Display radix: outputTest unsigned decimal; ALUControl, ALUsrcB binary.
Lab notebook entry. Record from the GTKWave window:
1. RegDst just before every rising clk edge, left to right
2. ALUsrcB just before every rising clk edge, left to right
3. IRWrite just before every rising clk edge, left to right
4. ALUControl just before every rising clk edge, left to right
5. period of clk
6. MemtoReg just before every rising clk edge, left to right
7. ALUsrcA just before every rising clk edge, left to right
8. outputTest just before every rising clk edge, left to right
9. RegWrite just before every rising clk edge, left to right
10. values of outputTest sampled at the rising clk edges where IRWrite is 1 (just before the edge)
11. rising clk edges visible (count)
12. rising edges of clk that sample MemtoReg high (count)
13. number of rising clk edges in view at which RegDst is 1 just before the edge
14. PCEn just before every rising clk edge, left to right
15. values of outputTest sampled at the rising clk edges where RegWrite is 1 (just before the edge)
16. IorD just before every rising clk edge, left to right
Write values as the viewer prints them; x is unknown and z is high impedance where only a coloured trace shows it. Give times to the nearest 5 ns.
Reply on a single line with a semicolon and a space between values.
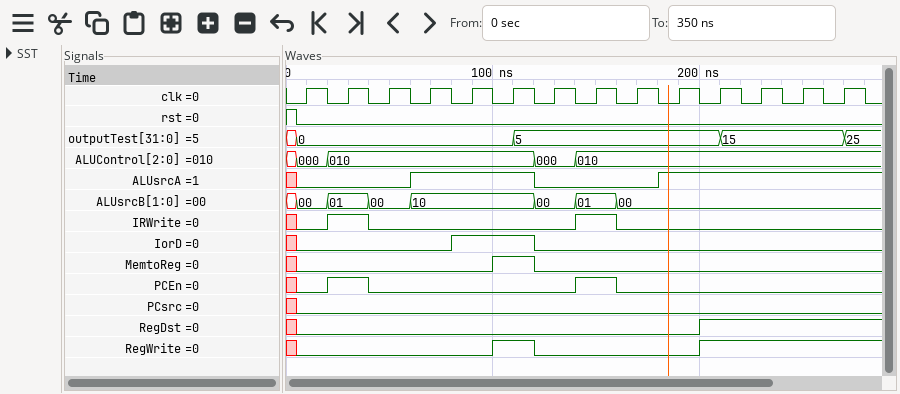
0 0 0 0 0 0 0 0 0 0 1 1 1 1; 00, 01, 00, 10, 10, 10, 00, 01, 00, 00, 00, 00, 00, 00; 0 1 0 0 0 0 0 1 0 0 0 0 0 0; 000, 010, 010, 010, 010, 010, 000, 010, 010, 010, 010, 010, 010, 010; 20 ns; 0 0 0 0 0 1 0 0 0 0 0 0 0 0; 0 0 0 1 1 1 0 0 0 1 1 1 1 1; 0, 0, 0, 0, 0, 0, 5, 5, 5, 5, 5, 15, 15, 15; 0 0 0 0 0 1 0 0 0 0 1 1 1 1; 0, 5; 14; 1; 4; 0 1 0 0 0 0 0 1 0 0 0 0 0 0; 0, 5, 15, 15, 15; 0 0 0 0 1 1 0 0 0 0 0 0 0 0
